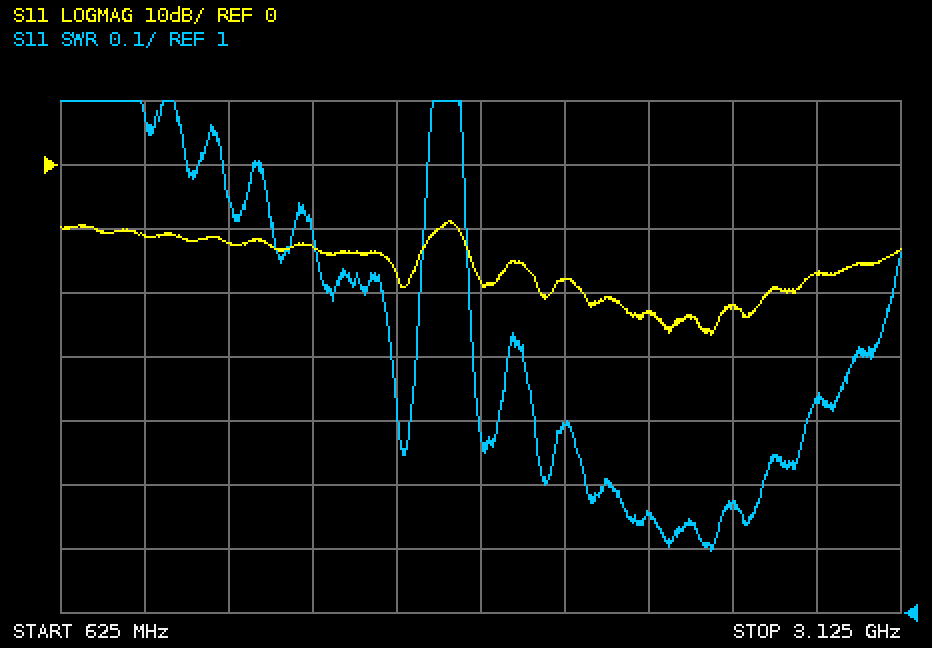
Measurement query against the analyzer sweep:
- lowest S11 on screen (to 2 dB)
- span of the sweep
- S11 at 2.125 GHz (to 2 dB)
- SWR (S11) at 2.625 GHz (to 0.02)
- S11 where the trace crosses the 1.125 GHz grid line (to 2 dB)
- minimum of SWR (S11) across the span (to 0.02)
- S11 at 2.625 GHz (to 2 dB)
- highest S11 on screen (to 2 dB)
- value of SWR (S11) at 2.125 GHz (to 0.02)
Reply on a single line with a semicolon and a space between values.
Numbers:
-26 dB; 2.5 GHz; -18 dB; 1.18; -12 dB; 1.10; -22 dB; -8 dB; 1.30
